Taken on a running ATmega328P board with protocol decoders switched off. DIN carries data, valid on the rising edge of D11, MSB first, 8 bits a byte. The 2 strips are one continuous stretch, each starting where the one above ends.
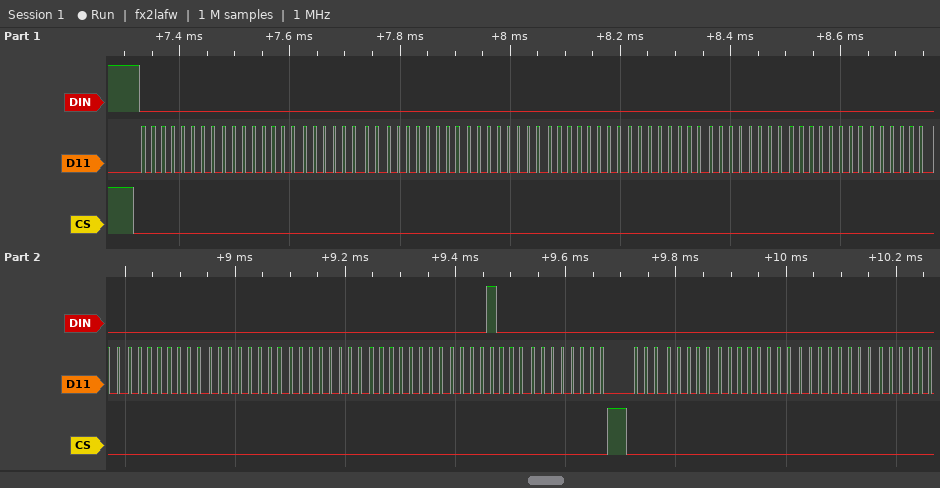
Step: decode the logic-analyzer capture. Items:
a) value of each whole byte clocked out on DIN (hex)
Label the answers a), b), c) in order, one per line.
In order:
a) 00 00 00 00 00 00 00 00 00 00 00 00 00 00 08 00 00 00 00
